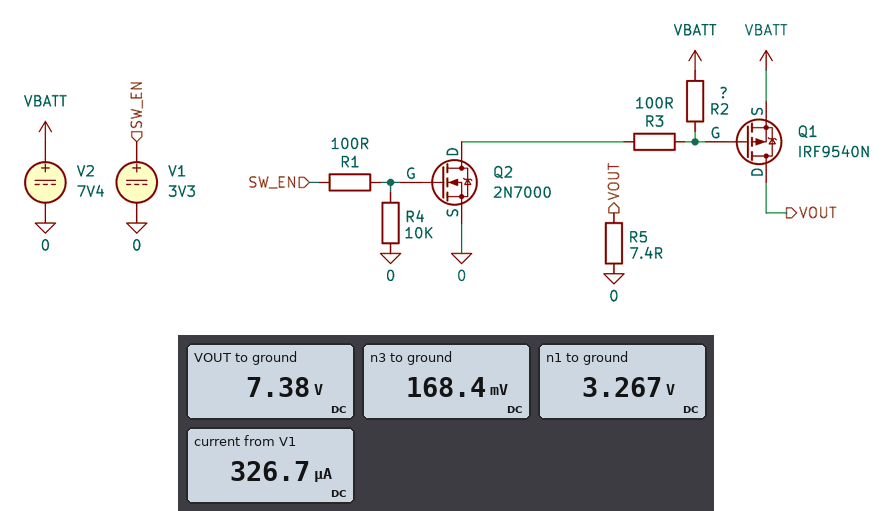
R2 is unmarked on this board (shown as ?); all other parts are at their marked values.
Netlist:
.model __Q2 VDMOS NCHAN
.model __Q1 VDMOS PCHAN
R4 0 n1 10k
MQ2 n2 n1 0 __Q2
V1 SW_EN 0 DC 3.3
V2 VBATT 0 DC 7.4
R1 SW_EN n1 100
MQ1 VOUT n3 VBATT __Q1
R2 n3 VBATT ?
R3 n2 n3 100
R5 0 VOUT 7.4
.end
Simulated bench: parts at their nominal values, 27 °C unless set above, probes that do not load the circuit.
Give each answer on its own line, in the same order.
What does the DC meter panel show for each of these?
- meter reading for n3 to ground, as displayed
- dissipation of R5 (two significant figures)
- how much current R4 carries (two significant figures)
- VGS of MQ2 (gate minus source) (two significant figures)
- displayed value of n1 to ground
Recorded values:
168.4 mV
7.4 W
330 µA
3.3 V
3.267 V
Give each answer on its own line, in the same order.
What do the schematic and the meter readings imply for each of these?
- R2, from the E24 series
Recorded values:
4.3 kΩ
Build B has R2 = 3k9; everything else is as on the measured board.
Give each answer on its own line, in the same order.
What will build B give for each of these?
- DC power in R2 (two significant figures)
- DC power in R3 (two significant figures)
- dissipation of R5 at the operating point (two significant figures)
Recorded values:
13 mW
340 µW
7.4 W
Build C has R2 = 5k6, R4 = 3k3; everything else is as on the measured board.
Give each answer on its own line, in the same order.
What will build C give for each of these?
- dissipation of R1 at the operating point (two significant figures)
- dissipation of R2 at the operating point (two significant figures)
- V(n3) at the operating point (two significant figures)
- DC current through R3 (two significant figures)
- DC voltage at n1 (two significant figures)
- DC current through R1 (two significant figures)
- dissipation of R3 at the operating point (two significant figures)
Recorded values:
94 µW
9.4 mW
130 mV
1.3 mA
3.2 V
970 µA
170 µW
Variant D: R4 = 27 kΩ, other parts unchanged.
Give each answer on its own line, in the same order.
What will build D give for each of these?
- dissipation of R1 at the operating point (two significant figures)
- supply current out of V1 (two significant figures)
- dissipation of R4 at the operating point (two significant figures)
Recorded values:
1.5 µW
120 µA
400 µW
